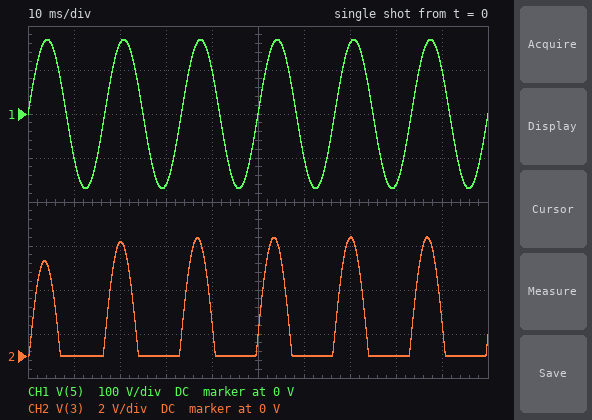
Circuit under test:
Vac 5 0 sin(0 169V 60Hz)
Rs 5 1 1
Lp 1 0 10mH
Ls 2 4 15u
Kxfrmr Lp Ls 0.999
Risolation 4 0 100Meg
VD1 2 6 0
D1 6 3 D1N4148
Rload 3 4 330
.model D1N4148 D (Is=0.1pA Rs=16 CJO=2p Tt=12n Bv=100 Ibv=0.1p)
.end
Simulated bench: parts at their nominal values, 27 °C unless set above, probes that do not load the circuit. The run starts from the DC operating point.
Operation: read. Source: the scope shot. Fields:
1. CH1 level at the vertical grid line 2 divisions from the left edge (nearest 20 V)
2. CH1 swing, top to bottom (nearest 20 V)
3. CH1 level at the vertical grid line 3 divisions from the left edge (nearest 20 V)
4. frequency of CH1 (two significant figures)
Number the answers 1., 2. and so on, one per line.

1. 160 V
2. 340 V
3. -160 V
4. 60 Hz
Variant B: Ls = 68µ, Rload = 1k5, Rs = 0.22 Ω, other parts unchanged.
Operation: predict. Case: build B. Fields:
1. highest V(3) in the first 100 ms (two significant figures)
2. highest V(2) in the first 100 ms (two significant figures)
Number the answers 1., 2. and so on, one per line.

1. 13 V
2. 14 V
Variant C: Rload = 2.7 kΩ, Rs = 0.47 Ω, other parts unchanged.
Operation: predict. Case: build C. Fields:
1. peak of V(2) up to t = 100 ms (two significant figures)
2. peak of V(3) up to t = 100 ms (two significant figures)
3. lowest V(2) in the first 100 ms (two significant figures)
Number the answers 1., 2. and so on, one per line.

1. 6.5 V
2. 5.8 V
3. -6.9 V
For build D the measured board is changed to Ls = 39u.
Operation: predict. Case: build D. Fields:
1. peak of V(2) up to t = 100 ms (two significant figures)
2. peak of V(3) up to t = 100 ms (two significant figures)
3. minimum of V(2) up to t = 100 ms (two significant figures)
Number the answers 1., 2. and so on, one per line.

1. 10 V
2. 9.1 V
3. -11 V
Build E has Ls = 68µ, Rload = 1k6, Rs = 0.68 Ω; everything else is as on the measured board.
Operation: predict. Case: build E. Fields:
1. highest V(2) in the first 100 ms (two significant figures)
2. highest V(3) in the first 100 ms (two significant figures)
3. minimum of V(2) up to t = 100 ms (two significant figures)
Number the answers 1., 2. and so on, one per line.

1. 14 V
2. 13 V
3. -15 V
